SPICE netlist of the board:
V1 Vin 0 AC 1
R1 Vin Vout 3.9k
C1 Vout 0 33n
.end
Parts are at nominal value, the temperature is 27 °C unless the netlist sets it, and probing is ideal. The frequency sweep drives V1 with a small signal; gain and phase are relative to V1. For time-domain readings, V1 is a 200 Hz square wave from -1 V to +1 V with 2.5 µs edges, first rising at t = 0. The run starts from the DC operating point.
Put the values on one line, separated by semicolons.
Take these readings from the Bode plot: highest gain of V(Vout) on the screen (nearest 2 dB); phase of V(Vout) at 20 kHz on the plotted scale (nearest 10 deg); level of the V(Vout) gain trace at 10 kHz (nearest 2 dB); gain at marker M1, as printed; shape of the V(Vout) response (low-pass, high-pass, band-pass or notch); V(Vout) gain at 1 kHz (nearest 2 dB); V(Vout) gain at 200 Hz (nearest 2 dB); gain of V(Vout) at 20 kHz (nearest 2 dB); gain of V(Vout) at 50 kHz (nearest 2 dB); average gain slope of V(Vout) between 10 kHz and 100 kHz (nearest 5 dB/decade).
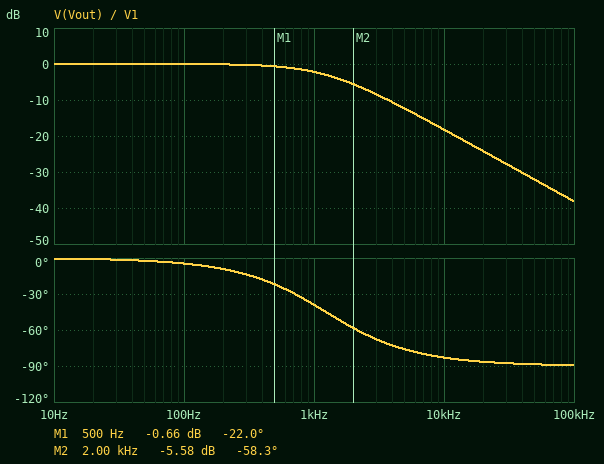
0 dB; -90 deg; -18 dB; -0.66 dB; low-pass; -2 dB; 0 dB; -24 dB; -32 dB; -20 dB/decade
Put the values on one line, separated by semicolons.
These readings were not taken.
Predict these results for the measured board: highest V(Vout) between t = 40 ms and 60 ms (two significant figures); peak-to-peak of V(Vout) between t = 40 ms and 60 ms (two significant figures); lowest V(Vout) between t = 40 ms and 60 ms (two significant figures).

1.0 V; 2.0 V; -1.0 V
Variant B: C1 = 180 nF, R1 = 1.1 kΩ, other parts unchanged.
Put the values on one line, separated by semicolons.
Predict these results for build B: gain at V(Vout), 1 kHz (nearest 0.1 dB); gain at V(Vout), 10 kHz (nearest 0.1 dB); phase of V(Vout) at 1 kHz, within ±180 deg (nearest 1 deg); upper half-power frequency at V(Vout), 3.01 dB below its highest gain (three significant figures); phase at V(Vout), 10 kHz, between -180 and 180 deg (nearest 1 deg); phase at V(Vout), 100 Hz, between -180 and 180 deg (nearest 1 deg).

-4.1 dB; -21.9 dB; -51 deg; 804 Hz; -85 deg; -7 deg
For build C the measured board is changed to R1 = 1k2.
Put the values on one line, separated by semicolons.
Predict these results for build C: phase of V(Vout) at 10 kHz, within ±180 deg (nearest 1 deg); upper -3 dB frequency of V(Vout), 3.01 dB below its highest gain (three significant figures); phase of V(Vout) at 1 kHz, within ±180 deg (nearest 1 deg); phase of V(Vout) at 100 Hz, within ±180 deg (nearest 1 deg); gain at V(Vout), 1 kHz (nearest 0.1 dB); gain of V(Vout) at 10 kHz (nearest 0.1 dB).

-68 deg; 4.02 kHz; -14 deg; -1 deg; -0.3 dB; -8.6 dB
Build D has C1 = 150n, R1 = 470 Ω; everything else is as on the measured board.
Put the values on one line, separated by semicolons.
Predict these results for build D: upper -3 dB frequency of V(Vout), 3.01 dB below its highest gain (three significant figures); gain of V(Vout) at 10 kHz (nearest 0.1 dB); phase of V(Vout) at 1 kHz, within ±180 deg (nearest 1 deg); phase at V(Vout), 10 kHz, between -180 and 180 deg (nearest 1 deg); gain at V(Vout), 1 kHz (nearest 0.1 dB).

2.26 kHz; -13.1 dB; -24 deg; -77 deg; -0.8 dB
